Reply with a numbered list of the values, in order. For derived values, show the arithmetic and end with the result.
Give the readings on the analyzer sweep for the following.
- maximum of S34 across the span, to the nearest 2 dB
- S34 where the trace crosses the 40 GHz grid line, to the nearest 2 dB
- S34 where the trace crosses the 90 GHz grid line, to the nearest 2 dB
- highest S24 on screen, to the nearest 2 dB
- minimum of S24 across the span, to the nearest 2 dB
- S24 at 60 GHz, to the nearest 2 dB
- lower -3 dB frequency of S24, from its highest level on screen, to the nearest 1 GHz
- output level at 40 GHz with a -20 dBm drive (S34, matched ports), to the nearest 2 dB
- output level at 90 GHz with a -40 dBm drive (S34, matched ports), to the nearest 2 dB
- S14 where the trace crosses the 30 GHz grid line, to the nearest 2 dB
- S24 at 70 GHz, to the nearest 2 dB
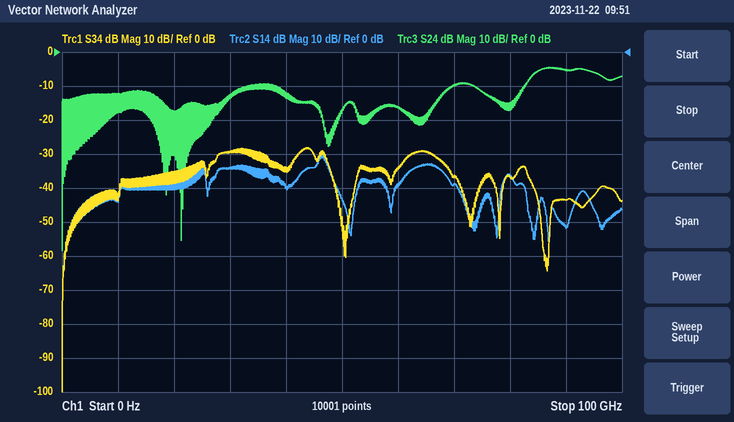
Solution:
1. -28 dB
2. -34 dB
3. -44 dB
4. -4 dB
5. -58 dB
6. -16 dB
7. 84 GHz
8. -20 dBm + (-34 dB) = -54 dBm
9. -40 dBm + (-44 dB) = -84 dBm
10. -34 dB
11. -10 dB
